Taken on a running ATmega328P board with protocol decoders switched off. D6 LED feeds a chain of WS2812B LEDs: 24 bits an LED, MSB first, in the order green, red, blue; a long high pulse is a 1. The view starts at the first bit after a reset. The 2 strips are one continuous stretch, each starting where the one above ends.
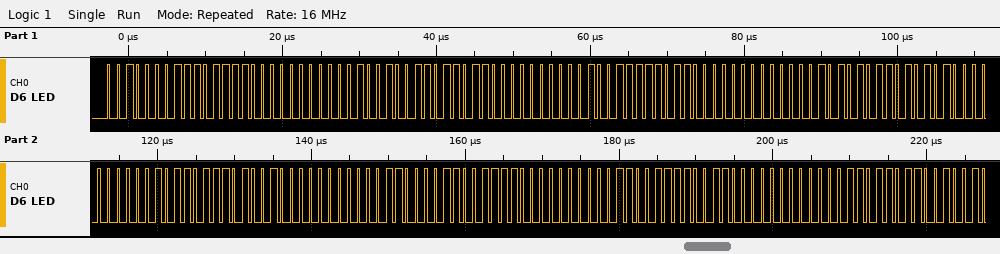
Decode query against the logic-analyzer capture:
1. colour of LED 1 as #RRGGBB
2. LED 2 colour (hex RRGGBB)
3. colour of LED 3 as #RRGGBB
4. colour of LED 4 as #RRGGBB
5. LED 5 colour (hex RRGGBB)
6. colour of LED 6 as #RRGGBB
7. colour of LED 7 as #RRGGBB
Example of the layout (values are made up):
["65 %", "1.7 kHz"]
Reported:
["#DE2100", "#DB2400", "#D82700", "#D52A00", "#D22D00", "#CF3000", "#CC3300"]
